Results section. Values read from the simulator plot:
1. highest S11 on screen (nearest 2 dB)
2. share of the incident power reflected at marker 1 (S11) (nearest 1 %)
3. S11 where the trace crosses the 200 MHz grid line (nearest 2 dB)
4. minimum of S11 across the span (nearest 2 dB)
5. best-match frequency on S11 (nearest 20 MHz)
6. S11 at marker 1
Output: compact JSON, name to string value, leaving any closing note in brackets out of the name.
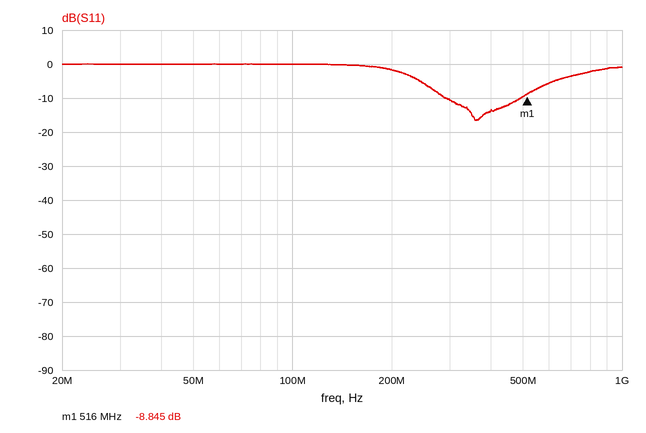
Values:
{"highest S11 on screen": "0 dB", "share of the incident power reflected at marker 1 (S11)": "13 %", "S11 where the trace crosses the 200 MHz grid line": "-2 dB", "minimum of S11 across the span": "-16 dB", "best-match frequency on S11": "360 MHz", "S11 at marker 1": "-8.845 dB"}
